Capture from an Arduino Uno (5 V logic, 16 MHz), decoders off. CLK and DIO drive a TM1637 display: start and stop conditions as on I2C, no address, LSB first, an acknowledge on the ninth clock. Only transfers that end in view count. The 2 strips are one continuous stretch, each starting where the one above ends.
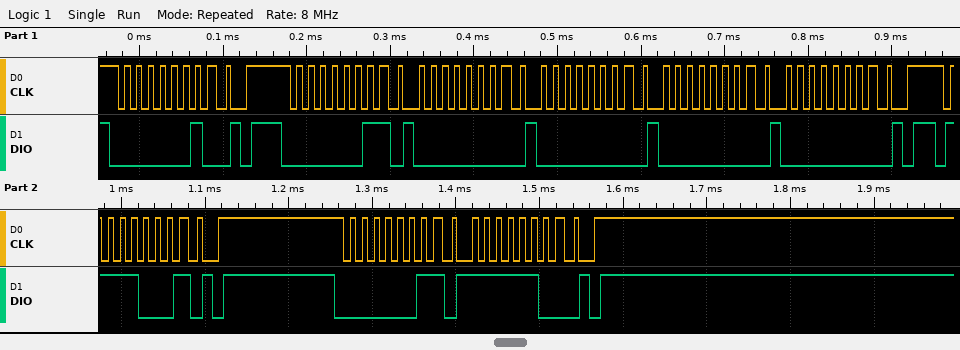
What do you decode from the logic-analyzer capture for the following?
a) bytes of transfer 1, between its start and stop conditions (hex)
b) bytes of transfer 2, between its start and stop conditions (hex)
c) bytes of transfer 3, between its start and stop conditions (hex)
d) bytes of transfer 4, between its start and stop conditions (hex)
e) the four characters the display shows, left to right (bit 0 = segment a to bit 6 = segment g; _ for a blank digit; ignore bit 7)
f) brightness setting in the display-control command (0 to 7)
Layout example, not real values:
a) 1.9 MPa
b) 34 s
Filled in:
a) 40
b) C0 00 00 00 00
c) 8F
d) C0 3F
e) 0___
f) 7
